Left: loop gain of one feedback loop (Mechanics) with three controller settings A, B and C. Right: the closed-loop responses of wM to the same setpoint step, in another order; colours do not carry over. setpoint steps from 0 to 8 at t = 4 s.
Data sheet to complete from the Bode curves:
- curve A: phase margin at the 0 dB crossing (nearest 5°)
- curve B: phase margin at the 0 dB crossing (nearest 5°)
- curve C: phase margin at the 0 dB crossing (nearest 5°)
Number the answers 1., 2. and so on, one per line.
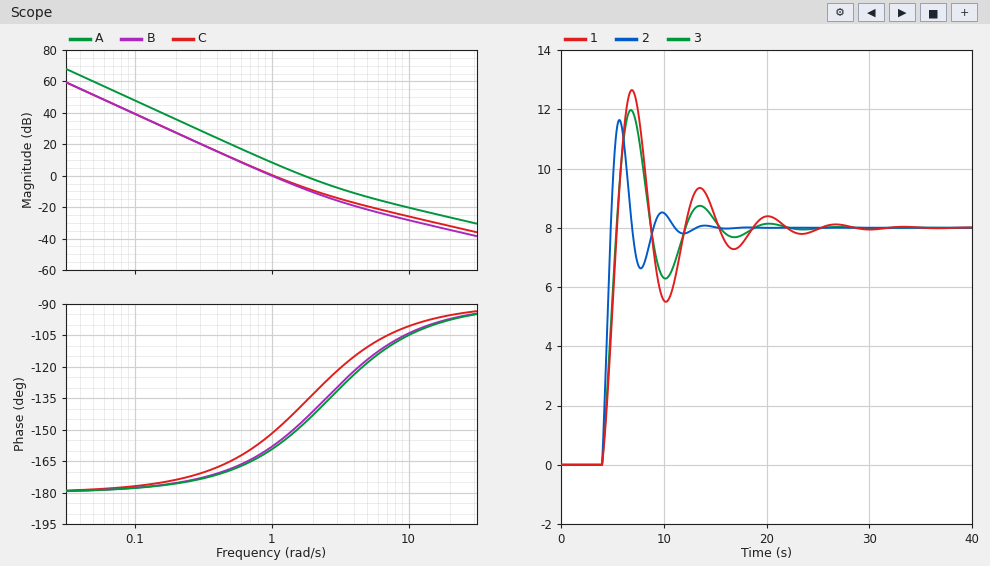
1. 35°
2. 20°
3. 30°
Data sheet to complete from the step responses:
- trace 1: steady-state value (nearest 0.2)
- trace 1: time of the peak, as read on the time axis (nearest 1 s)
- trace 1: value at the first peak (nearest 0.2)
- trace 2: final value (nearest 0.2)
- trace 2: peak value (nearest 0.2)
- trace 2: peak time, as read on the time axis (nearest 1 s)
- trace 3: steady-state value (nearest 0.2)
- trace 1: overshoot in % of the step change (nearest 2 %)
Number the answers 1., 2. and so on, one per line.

1. 8.0
2. 7 s
3. 12.6
4. 8.0
5. 11.6
6. 6 s
7. 8.0
8. 58 %
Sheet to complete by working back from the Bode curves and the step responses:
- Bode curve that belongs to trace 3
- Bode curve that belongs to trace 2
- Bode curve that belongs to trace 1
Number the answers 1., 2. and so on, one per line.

1. C
2. A
3. B
